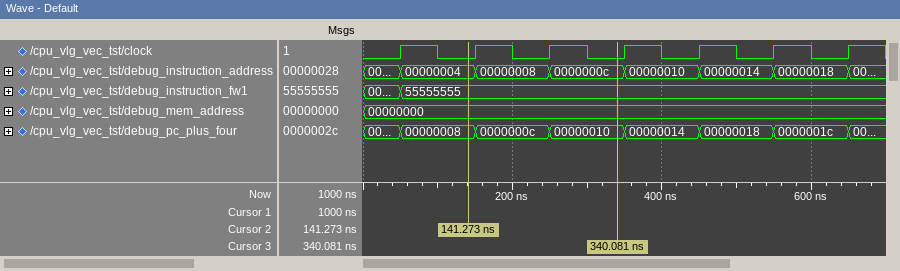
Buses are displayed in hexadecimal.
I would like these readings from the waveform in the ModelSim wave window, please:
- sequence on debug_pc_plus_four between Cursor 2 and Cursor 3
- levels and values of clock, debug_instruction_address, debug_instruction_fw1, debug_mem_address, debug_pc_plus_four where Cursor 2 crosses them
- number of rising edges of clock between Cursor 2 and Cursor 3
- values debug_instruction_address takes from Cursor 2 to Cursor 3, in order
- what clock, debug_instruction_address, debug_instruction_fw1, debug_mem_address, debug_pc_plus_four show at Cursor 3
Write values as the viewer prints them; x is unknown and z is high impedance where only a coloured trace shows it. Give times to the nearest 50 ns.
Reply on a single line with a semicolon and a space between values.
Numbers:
00000008, 0000000c, 00000010; clock=0, debug_instruction_address=00000004, debug_instruction_fw1=55555555, debug_mem_address=00000000, debug_pc_plus_four=00000008; 2; 00000004, 00000008, 0000000c; clock=0, debug_instruction_address=0000000c, debug_instruction_fw1=55555555, debug_mem_address=00000000, debug_pc_plus_four=00000010
